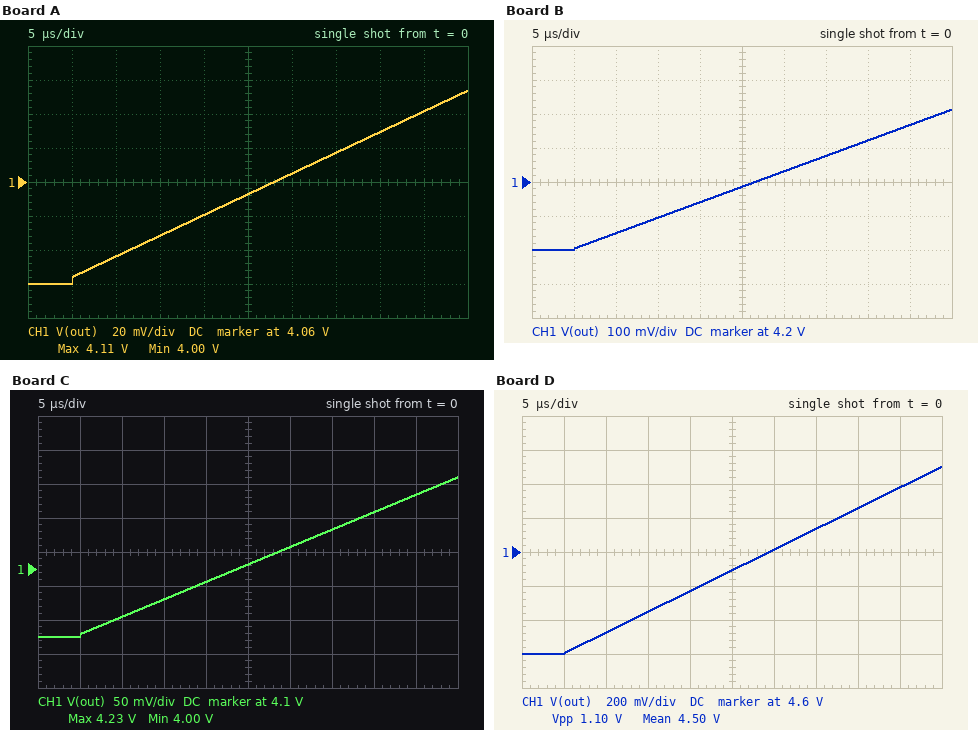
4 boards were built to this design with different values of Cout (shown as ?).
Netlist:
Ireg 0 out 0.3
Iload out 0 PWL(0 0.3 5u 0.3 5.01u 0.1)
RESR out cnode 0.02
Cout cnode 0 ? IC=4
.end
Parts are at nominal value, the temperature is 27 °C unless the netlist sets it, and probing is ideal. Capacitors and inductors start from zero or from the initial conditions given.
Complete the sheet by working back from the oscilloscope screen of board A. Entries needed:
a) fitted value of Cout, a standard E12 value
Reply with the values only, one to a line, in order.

82 µF
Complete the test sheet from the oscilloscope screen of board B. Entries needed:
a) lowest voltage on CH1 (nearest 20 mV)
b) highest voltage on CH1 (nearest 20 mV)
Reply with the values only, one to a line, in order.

4.00 V
4.42 V
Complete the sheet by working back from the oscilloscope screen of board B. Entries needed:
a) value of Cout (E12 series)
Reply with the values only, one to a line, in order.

22 µF
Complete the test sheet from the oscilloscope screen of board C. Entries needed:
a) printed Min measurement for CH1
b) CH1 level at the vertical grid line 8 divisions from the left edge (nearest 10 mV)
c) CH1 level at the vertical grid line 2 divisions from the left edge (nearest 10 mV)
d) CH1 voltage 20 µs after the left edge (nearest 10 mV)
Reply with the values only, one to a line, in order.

4.00 V
4.18 V
4.03 V
4.08 V
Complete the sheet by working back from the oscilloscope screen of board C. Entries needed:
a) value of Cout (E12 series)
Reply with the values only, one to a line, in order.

39 µF
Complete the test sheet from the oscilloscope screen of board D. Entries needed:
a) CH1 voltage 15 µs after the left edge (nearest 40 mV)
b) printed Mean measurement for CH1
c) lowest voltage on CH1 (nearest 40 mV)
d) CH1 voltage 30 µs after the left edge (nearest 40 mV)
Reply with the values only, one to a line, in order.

4.24 V
4.50 V
4.00 V
4.60 V
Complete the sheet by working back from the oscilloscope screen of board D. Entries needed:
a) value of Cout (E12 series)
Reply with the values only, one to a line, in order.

8.2 µF
